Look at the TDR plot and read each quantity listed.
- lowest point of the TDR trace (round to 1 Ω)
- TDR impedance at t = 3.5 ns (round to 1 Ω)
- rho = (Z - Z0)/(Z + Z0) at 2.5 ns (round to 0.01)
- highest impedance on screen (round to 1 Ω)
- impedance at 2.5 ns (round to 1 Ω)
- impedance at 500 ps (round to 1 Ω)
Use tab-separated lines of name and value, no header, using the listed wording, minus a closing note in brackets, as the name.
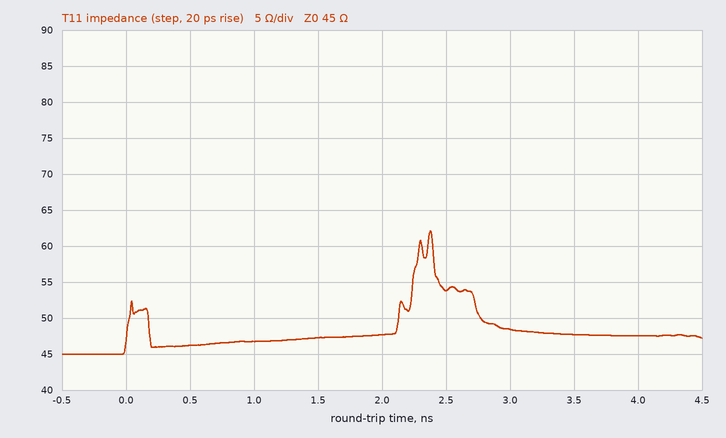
lowest point of the TDR trace	45 Ω
TDR impedance at t = 3.5 ns	48 Ω
rho = (Z - Z0)/(Z + Z0) at 2.5 ns	+0.09
highest impedance on screen	62 Ω
impedance at 2.5 ns	54 Ω
impedance at 500 ps	46 Ω
